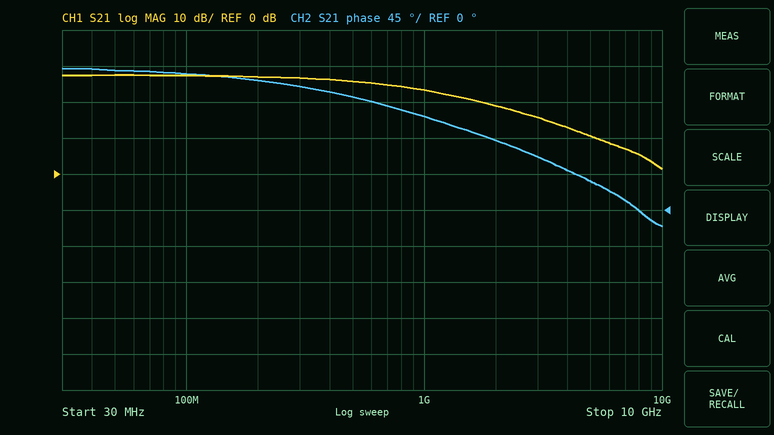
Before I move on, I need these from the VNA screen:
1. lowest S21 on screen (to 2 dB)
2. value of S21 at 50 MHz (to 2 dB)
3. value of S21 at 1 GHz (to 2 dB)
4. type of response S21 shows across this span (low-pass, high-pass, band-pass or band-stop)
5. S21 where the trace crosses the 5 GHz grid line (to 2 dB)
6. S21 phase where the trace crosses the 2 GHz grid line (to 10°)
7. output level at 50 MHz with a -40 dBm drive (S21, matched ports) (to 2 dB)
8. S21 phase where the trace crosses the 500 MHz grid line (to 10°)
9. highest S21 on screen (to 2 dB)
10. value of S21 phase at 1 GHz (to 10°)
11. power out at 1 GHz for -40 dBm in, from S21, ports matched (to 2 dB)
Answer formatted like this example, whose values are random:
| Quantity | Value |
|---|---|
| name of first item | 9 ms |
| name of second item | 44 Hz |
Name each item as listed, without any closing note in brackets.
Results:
| Quantity | Value |
|---|---|
| lowest S21 on screen | 2 dB |
| value of S21 at 50 MHz | 28 dB |
| value of S21 at 1 GHz | 24 dB |
| type of response S21 shows across this span | low-pass |
| S21 where the trace crosses the 5 GHz grid line | 10 dB |
| S21 phase where the trace crosses the 2 GHz grid line | 90° |
| output level at 50 MHz with a -40 dBm drive (S21, matched ports) | -12 dBm |
| S21 phase where the trace crosses the 500 MHz grid line | 140° |
| highest S21 on screen | 28 dB |
| value of S21 phase at 1 GHz | 120° |
| power out at 1 GHz for -40 dBm in, from S21, ports matched | -16 dBm |
